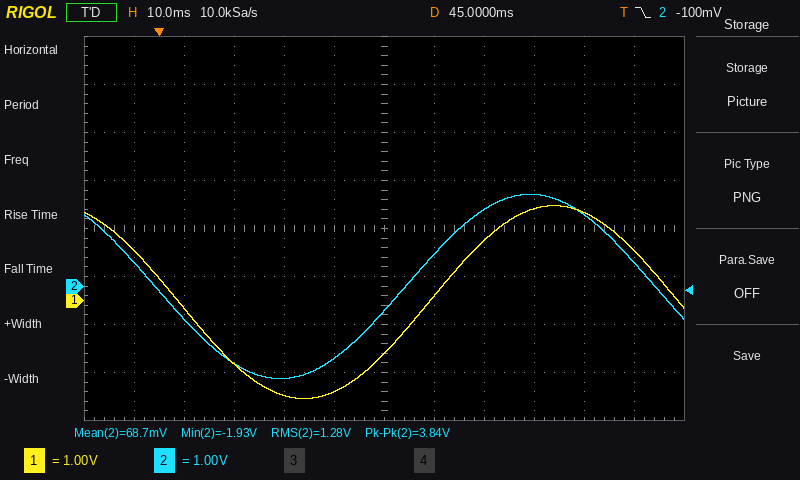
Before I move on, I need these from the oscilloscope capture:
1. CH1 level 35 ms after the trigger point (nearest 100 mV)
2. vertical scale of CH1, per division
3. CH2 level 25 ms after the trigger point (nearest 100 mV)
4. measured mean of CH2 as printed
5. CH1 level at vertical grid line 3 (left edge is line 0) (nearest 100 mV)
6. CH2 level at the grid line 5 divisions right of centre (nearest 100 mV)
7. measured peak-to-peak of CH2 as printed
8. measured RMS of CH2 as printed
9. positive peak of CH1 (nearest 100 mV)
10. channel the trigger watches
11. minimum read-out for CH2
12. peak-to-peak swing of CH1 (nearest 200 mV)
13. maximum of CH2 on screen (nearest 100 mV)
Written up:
-1.9 V
1 V
-1.9 V
68.7 mV
-1.3 V
500 mV
3.84 V
1.28 V
2.0 V
CH2
-1.93 V
4.0 V
1.9 V
